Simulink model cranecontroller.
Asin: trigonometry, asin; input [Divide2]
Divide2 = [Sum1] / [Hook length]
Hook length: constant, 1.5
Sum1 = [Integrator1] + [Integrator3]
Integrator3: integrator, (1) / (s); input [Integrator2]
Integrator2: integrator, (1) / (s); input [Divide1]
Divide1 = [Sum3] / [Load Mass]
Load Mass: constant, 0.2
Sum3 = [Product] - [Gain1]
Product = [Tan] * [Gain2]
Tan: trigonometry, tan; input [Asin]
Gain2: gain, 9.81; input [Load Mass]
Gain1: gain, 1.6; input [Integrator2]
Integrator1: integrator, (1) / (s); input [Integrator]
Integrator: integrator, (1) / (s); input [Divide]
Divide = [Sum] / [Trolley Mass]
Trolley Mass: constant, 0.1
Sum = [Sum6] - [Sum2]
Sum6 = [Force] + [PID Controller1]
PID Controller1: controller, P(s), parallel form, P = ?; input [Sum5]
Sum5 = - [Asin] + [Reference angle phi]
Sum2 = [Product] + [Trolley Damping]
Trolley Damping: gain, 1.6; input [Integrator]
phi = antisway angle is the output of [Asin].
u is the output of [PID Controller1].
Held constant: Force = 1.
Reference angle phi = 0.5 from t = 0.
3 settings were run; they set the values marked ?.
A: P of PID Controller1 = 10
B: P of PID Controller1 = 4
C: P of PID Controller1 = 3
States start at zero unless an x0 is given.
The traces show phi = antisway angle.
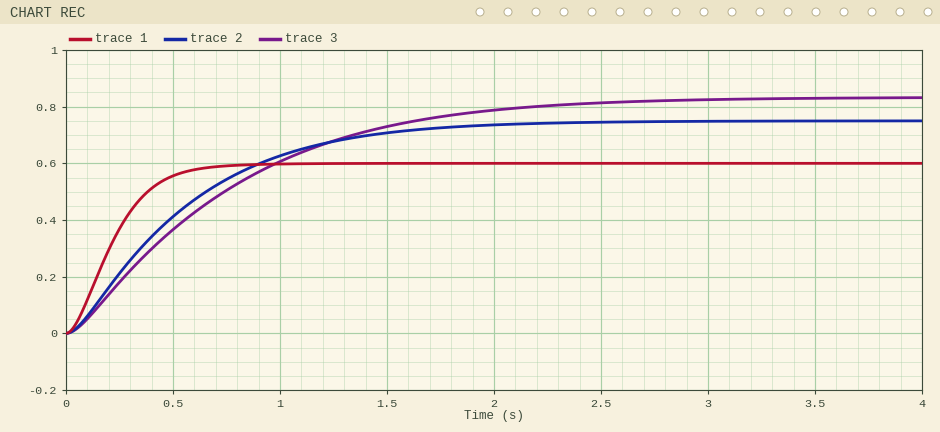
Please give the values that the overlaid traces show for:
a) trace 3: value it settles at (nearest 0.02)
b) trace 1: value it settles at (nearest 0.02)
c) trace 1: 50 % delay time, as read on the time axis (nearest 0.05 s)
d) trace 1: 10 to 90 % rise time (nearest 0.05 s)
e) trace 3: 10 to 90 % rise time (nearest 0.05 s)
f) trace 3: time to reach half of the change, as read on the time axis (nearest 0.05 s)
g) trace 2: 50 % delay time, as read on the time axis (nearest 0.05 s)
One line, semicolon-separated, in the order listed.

0.84; 0.60; 0.20 s; 0.40 s; 1.50 s; 0.60 s; 0.45 s
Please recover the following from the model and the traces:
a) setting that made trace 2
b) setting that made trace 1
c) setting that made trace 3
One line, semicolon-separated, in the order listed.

B; A; C
